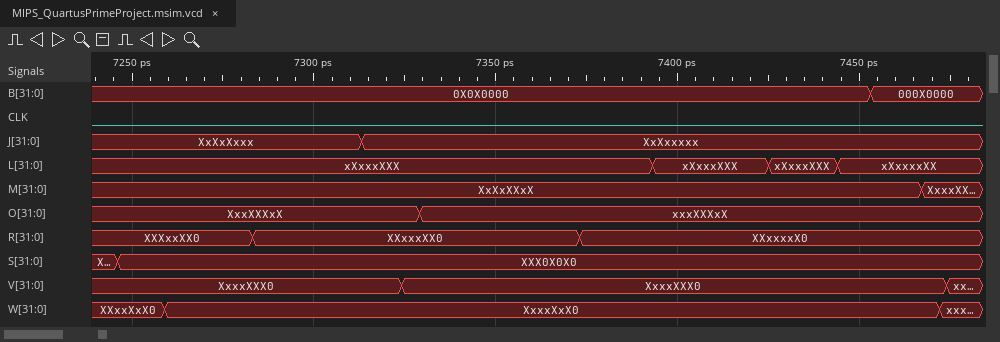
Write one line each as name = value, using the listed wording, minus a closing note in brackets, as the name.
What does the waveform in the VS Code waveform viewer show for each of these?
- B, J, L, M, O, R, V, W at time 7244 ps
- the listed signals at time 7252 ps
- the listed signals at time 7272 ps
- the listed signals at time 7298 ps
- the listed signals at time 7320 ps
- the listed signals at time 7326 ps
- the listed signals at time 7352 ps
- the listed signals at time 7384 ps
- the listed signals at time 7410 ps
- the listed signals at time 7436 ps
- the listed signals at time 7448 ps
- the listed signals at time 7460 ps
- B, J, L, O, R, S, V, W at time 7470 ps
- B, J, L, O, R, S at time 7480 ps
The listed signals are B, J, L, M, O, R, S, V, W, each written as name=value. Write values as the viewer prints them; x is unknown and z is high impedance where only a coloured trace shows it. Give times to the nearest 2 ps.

B, J, L, M, O, R, V, W at time 7244 ps = B=0X0X0000, J=XxXxXxxx, L=xXxxxXXX, M=XxXxXXxX, O=XxxXXXxX, R=XXXxxXX0, V=XxxxXXX0, W=XXxxXxX0
the listed signals at time 7252 ps = B=0X0X0000, J=XxXxXxxx, L=xXxxxXXX, M=XxXxXXxX, O=XxxXXXxX, R=XXXxxXX0, S=XXX0X0X0, V=XxxxXXX0, W=XXxxXxX0
the listed signals at time 7272 ps = B=0X0X0000, J=XxXxXxxx, L=xXxxxXXX, M=XxXxXXxX, O=XxxXXXxX, R=XXXxxXX0, S=XXX0X0X0, V=XxxxXXX0, W=XxxxXxX0
the listed signals at time 7298 ps = B=0X0X0000, J=XxXxXxxx, L=xXxxxXXX, M=XxXxXXxX, O=XxxXXXxX, R=XXxxxXX0, S=XXX0X0X0, V=XxxxXXX0, W=XxxxXxX0
the listed signals at time 7320 ps = B=0X0X0000, J=XxXxxxxx, L=xXxxxXXX, M=XxXxXXxX, O=XxxXXXxX, R=XXxxxXX0, S=XXX0X0X0, V=XxxxXXX0, W=XxxxXxX0
the listed signals at time 7326 ps = B=0X0X0000, J=XxXxxxxx, L=xXxxxXXX, M=XxXxXXxX, O=XxxXXXxX, R=XXxxxXX0, S=XXX0X0X0, V=XxxxXXX0, W=XxxxXxX0
the listed signals at time 7352 ps = B=0X0X0000, J=XxXxxxxx, L=xXxxxXXX, M=XxXxXXxX, O=xxxXXXxX, R=XXxxxXX0, S=XXX0X0X0, V=XxxxXXX0, W=XxxxXxX0
the listed signals at time 7384 ps = B=0X0X0000, J=XxXxxxxx, L=xXxxxXXX, M=XxXxXXxX, O=xxxXXXxX, R=XXxxxxX0, S=XXX0X0X0, V=XxxxXXX0, W=XxxxXxX0
the listed signals at time 7410 ps = B=0X0X0000, J=XxXxxxxx, L=xXxxxXXX, M=XxXxXXxX, O=xxxXXXxX, R=XXxxxxX0, S=XXX0X0X0, V=XxxxXXX0, W=XxxxXxX0
the listed signals at time 7436 ps = B=0X0X0000, J=XxXxxxxx, L=xXxxxXXX, M=XxXxXXxX, O=xxxXXXxX, R=XXxxxxX0, S=XXX0X0X0, V=XxxxXXX0, W=XxxxXxX0
the listed signals at time 7448 ps = B=0X0X0000, J=XxXxxxxx, L=xXxxxxXX, M=XxXxXXxX, O=xxxXXXxX, R=XXxxxxX0, S=XXX0X0X0, V=XxxxXXX0, W=XxxxXxX0
the listed signals at time 7460 ps = B=000X0000, J=XxXxxxxx, L=xXxxxxXX, M=XxXxXXxX, O=xxxXXXxX, R=XXxxxxX0, S=XXX0X0X0, V=XxxxXXX0, W=XxxxXxX0
B, J, L, O, R, S, V, W at time 7470 ps = B=000X0000, J=XxXxxxxx, L=xXxxxxXX, O=xxxXXXxX, R=XXxxxxX0, S=XXX0X0X0, V=XxxxXXX0, W=XxxxXxX0
B, J, L, O, R, S at time 7480 ps = B=000X0000, J=XxXxxxxx, L=xXxxxxXX, O=xxxXXXxX, R=XXxxxxX0, S=XXX0X0X0
